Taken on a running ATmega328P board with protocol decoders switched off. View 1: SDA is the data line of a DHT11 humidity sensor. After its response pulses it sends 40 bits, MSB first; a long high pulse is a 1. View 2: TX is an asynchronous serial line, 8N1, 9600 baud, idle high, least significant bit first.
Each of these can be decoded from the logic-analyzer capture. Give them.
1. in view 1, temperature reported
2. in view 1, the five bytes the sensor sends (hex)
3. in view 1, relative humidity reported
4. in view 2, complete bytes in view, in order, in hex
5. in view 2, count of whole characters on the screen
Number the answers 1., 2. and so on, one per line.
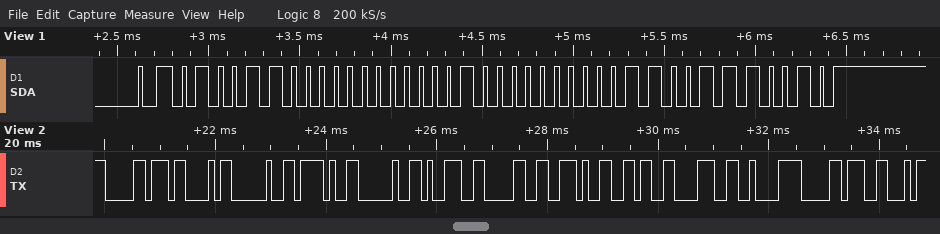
1. 32.6 °C
2. 4C 00 20 06 72
3. 76 %
4. B0 43 20 2F 20 39 30 2E 36 38 C2 B0 46
5. 13
